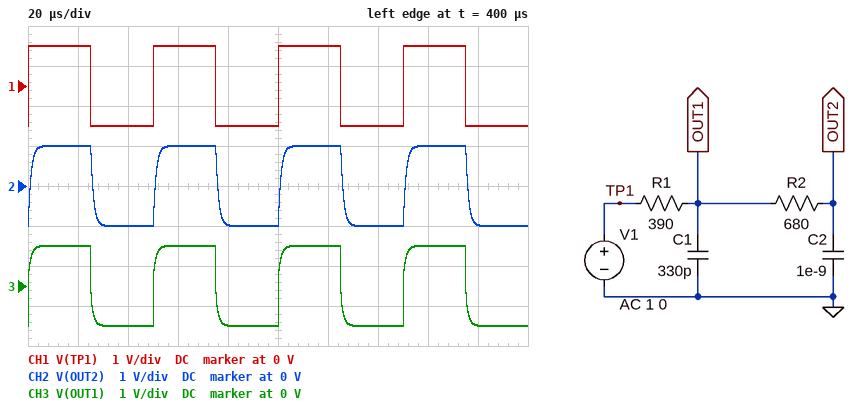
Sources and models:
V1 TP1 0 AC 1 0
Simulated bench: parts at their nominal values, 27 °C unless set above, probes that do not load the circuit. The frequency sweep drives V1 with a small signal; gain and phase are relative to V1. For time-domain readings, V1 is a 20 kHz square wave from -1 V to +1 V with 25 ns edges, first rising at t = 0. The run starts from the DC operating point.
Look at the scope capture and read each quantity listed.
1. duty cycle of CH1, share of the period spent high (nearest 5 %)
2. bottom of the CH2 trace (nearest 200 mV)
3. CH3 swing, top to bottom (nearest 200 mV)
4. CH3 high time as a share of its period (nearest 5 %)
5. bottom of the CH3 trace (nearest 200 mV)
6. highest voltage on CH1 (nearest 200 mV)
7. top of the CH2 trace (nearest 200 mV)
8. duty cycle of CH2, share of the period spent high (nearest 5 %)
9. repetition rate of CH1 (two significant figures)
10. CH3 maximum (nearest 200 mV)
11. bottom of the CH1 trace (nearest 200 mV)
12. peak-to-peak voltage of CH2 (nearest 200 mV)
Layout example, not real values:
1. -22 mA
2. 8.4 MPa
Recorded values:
1. 50 %
2. -1.0 V
3. 2.0 V
4. 50 %
5. -1.0 V
6. 1.0 V
7. 1.0 V
8. 50 %
9. 20 kHz
10. 1.0 V
11. -1.0 V
12. 2.0 V
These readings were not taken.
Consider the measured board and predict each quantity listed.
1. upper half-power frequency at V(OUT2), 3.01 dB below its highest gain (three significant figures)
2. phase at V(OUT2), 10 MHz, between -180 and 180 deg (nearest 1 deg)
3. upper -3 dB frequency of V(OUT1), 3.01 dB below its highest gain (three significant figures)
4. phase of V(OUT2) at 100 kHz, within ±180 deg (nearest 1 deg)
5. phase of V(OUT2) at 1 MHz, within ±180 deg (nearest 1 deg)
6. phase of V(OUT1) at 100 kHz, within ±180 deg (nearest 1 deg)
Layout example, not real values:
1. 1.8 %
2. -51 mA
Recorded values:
1. 141 kHz
2. -168 deg
3. 266 kHz
4. -38 deg
5. -108 deg
6. -15 deg
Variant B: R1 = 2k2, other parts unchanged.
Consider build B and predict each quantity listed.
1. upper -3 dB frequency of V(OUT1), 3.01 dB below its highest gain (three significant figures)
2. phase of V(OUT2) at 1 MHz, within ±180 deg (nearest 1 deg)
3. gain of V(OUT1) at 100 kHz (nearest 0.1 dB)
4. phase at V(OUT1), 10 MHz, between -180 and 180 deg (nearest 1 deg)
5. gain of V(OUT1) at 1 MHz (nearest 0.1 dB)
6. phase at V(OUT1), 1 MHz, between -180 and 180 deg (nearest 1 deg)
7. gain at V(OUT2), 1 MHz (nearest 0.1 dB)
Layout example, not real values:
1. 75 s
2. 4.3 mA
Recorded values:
1. 47.7 kHz
2. -129 deg
3. -6.9 dB
4. -85 deg
5. -16.5 dB
6. -52 deg
7. -29.3 dB
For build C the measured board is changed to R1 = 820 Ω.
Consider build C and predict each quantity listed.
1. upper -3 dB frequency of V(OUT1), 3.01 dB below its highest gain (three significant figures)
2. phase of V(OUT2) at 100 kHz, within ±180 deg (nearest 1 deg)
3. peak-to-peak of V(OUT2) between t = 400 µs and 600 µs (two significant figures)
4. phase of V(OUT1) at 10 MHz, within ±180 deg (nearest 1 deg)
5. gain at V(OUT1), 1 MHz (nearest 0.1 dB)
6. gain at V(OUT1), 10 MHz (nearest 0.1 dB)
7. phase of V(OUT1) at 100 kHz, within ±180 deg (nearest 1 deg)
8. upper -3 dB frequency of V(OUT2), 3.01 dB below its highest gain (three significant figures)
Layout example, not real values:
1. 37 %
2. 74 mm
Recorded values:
1. 117 kHz
2. -50 deg
3. 2.0 V
4. -83 deg
5. -9.3 dB
6. -24.7 dB
7. -27 deg
8. 95.5 kHz
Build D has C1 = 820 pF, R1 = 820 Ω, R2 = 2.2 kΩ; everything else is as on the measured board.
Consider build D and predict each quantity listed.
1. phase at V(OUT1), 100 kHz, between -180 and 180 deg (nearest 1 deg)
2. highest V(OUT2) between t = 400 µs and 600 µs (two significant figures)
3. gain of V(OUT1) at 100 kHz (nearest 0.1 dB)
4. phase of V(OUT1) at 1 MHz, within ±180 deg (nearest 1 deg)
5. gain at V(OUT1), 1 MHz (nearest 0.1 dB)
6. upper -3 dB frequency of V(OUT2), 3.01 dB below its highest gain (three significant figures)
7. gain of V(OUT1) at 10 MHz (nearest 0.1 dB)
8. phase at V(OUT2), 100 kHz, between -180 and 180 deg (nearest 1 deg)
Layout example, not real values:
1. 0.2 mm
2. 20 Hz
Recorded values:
1. -26 deg
2. 1.0 V
3. -2.8 dB
4. -72 deg
5. -13.0 dB
6. 48.3 kHz
7. -32.5 dB
8. -80 deg
